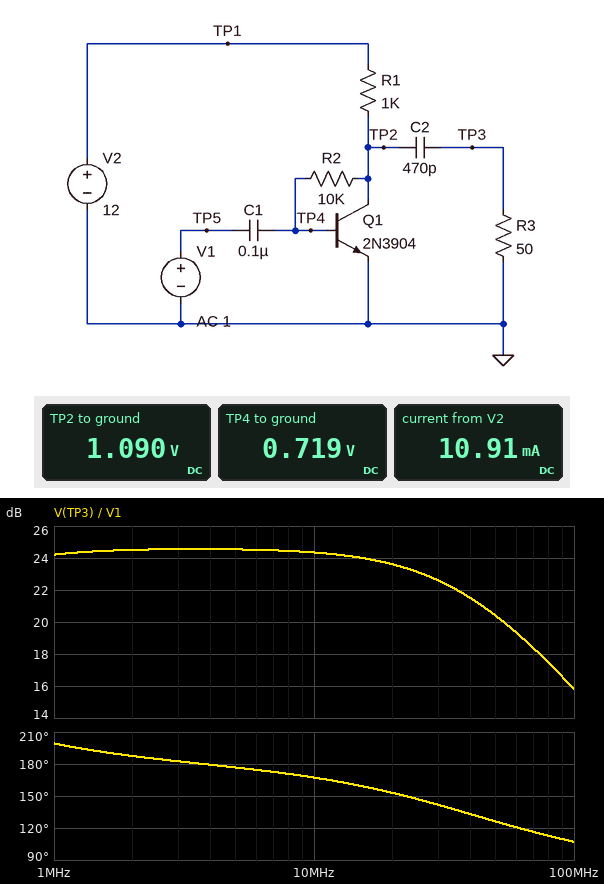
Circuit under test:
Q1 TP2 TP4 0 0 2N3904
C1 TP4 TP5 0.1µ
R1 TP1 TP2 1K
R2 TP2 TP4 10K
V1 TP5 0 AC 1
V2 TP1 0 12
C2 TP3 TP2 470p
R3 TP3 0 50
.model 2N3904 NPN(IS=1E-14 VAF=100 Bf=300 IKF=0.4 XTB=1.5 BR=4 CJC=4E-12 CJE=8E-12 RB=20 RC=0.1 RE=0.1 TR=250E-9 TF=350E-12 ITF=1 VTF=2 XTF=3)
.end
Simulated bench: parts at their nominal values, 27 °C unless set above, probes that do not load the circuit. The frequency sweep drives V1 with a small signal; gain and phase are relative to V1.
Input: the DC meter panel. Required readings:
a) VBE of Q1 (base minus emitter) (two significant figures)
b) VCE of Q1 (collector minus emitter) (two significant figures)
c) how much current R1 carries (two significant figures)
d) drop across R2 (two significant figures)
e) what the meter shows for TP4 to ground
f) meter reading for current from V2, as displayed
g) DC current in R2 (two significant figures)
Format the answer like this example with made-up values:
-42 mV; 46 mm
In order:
720 mV; 1.1 V; 11 mA; 370 mV; 0.719 V; 10.91 mA; 37 µA
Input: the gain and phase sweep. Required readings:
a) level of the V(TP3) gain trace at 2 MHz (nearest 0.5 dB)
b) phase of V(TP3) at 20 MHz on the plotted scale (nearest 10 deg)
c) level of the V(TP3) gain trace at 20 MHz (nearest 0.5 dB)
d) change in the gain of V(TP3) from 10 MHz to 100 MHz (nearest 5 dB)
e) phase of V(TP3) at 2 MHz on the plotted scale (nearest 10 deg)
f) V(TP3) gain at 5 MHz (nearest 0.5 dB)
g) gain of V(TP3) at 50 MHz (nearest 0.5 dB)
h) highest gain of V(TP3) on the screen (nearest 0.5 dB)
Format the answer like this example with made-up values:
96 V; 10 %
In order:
24.5 dB; 150 deg; 23.5 dB; -10 dB; 190 deg; 24.5 dB; 20.5 dB; 24.5 dB
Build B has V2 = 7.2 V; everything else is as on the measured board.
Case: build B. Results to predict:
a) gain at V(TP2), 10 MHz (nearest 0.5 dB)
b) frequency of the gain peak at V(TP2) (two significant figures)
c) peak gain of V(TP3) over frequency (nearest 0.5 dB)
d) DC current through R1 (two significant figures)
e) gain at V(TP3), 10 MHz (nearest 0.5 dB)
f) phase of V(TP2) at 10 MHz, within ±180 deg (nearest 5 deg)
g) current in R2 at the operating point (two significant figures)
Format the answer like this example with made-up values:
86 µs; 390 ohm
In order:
22.0 dB; 110 kHz; 20.5 dB; 6.3 mA; 20.0 dB; 140 deg; 21 µA
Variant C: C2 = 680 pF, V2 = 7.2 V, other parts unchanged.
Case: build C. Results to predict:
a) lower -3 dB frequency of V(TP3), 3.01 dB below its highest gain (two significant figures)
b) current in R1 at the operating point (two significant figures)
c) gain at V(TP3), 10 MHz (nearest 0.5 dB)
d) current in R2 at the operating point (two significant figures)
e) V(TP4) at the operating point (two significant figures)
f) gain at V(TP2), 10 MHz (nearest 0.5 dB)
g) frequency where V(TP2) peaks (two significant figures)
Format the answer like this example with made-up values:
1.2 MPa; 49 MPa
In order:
220 kHz; 6.3 mA; 20.5 dB; 21 µA; 700 mV; 21.0 dB; 91 kHz
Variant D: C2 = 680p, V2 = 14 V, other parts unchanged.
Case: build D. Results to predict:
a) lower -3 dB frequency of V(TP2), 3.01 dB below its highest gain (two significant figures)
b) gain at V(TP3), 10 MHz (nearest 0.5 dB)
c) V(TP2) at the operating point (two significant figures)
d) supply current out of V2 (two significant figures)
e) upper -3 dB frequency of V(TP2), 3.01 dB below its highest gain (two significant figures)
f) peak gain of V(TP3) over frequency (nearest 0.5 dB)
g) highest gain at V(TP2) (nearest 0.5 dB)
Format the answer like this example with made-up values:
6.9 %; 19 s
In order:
49 kHz; 25.5 dB; 1.2 V; 13 mA; 320 kHz; 26.0 dB; 51.0 dB
